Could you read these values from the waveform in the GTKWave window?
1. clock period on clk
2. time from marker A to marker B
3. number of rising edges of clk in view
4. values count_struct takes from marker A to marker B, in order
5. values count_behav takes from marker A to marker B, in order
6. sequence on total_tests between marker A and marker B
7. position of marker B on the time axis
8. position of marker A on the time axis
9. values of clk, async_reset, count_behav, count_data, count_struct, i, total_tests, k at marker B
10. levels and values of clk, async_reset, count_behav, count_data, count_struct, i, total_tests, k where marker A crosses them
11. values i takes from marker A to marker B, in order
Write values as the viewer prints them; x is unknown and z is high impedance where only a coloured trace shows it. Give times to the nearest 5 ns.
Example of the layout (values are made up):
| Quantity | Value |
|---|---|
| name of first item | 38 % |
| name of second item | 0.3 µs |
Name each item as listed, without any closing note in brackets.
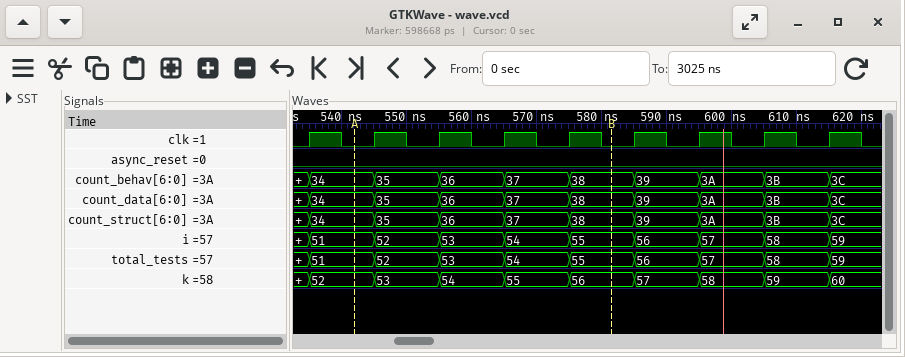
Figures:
| Quantity | Value |
|---|---|
| clock period on clk | 10 ns |
| time from marker A to marker B | 40 ns |
| number of rising edges of clk in view | 9 |
| values count_struct takes from marker A to marker B, in order | 34, 35, 36, 37, 38 |
| values count_behav takes from marker A to marker B, in order | 34, 35, 36, 37, 38 |
| sequence on total_tests between marker A and marker B | 51, 52, 53, 54, 55 |
| position of marker B on the time axis | 580 ns |
| position of marker A on the time axis | 540 ns |
| values of clk, async_reset, count_behav, count_data, count_struct, i, total_tests, k at marker B | clk=0, async_reset=0, count_behav=38, count_data=38, count_struct=38, i=55, total_tests=55, k=56 |
| levels and values of clk, async_reset, count_behav, count_data, count_struct, i, total_tests, k where marker A crosses them | clk=0, async_reset=0, count_behav=34, count_data=34, count_struct=34, i=51, total_tests=51, k=52 |
| values i takes from marker A to marker B, in order | 51, 52, 53, 54, 55 |
